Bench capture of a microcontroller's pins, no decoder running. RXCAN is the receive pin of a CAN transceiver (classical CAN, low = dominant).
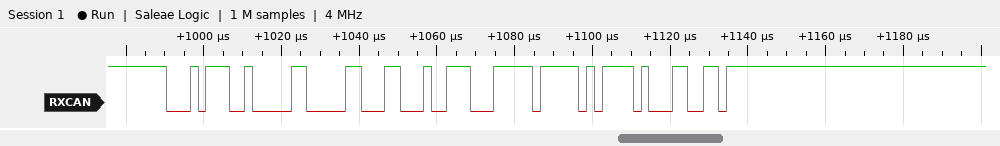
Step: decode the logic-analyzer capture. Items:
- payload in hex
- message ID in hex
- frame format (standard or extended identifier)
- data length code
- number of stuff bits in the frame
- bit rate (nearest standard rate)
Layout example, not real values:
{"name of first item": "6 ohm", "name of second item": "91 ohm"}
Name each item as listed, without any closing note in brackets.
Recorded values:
{"payload in hex": "11 89 C7 FF", "message ID in hex": "0x172", "frame format": "standard", "data length code": "4", "number of stuff bits in the frame": "4", "bit rate": "500 kbit/s"}
